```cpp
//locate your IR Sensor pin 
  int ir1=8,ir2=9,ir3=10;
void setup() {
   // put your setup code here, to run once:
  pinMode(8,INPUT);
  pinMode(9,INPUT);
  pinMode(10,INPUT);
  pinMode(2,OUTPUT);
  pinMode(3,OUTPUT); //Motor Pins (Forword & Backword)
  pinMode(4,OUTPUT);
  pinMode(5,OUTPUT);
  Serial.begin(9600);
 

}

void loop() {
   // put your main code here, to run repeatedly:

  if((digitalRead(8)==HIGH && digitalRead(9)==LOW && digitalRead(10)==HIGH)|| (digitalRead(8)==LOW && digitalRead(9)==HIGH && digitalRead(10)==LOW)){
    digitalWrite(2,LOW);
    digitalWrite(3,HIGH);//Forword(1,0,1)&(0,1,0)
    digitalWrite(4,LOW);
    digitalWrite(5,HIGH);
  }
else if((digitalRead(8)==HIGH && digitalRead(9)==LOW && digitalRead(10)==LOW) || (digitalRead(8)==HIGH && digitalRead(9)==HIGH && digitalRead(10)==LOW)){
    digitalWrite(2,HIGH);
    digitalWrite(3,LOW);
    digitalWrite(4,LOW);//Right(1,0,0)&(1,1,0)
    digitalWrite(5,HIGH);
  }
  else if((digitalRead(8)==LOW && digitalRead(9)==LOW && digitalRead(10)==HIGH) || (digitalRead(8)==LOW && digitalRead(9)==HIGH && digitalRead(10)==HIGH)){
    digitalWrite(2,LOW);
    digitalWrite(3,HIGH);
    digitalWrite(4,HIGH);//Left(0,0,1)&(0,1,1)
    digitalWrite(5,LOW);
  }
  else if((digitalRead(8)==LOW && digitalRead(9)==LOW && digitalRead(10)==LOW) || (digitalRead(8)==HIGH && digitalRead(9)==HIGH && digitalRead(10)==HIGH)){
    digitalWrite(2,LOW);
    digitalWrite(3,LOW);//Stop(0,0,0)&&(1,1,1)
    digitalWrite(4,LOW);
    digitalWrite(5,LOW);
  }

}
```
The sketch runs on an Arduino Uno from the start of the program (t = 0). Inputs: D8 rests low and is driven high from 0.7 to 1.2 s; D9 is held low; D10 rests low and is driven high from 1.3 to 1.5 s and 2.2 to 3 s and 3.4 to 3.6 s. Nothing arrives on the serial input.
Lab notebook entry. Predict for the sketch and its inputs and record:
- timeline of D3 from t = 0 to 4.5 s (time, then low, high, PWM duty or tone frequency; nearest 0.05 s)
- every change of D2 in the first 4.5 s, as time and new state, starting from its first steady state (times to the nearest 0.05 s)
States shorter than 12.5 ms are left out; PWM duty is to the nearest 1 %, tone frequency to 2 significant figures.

0 s low; 1.3 s high; 1.5 s low; 2.2 s high; 3 s low; 3.4 s high; 3.6 s low
0 s low; 0.7 s high; 1.2 s low
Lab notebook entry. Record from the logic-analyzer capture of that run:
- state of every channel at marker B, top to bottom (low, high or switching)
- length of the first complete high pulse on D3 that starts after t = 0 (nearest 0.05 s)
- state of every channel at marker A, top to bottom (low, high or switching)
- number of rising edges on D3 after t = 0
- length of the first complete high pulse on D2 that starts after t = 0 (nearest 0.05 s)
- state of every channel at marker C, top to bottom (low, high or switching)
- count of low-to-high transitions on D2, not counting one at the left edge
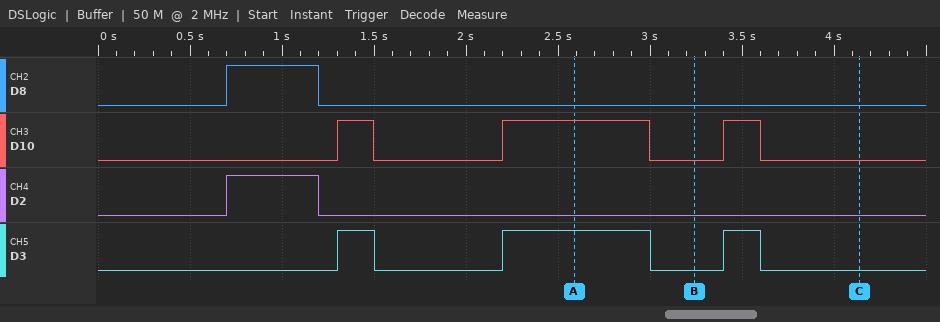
D8 low, D10 low, D2 low, D3 low
0.20 s
D8 low, D10 high, D2 low, D3 high
3
0.50 s
D8 low, D10 low, D2 low, D3 low
1
